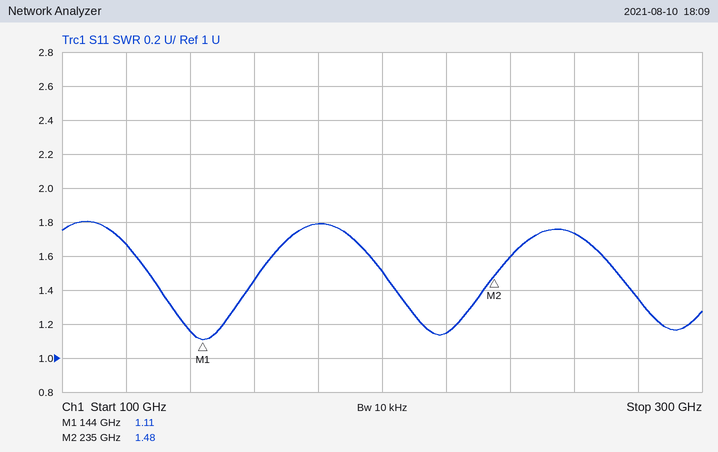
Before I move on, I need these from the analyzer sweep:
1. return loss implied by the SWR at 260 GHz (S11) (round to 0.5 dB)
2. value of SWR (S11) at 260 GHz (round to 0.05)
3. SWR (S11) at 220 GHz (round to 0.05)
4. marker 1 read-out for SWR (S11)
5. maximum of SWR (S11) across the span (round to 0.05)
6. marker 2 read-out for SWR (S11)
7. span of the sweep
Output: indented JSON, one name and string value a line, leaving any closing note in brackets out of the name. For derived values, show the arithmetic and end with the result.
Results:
{
  "return loss implied by the SWR at 260 GHz (S11)": "−20 log10((1.75 − 1)/(1.75 + 1)) ≈ 11.3 dB, so 11.5 dB to the nearest 0.5 dB",
  "value of SWR (S11) at 260 GHz": "1.75",
  "SWR (S11) at 220 GHz": "1.15",
  "marker 1 read-out for SWR": "1.11",
  "maximum of SWR (S11) across the span": "1.80",
  "marker 2 read-out for SWR": "1.48",
  "span of the sweep": "200 GHz"
}
